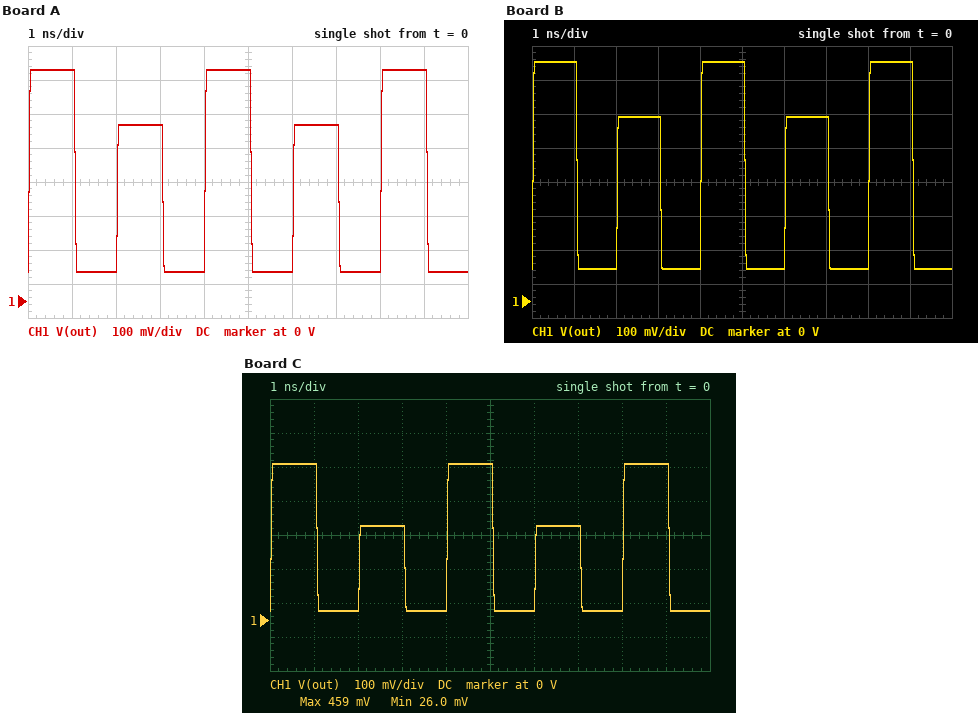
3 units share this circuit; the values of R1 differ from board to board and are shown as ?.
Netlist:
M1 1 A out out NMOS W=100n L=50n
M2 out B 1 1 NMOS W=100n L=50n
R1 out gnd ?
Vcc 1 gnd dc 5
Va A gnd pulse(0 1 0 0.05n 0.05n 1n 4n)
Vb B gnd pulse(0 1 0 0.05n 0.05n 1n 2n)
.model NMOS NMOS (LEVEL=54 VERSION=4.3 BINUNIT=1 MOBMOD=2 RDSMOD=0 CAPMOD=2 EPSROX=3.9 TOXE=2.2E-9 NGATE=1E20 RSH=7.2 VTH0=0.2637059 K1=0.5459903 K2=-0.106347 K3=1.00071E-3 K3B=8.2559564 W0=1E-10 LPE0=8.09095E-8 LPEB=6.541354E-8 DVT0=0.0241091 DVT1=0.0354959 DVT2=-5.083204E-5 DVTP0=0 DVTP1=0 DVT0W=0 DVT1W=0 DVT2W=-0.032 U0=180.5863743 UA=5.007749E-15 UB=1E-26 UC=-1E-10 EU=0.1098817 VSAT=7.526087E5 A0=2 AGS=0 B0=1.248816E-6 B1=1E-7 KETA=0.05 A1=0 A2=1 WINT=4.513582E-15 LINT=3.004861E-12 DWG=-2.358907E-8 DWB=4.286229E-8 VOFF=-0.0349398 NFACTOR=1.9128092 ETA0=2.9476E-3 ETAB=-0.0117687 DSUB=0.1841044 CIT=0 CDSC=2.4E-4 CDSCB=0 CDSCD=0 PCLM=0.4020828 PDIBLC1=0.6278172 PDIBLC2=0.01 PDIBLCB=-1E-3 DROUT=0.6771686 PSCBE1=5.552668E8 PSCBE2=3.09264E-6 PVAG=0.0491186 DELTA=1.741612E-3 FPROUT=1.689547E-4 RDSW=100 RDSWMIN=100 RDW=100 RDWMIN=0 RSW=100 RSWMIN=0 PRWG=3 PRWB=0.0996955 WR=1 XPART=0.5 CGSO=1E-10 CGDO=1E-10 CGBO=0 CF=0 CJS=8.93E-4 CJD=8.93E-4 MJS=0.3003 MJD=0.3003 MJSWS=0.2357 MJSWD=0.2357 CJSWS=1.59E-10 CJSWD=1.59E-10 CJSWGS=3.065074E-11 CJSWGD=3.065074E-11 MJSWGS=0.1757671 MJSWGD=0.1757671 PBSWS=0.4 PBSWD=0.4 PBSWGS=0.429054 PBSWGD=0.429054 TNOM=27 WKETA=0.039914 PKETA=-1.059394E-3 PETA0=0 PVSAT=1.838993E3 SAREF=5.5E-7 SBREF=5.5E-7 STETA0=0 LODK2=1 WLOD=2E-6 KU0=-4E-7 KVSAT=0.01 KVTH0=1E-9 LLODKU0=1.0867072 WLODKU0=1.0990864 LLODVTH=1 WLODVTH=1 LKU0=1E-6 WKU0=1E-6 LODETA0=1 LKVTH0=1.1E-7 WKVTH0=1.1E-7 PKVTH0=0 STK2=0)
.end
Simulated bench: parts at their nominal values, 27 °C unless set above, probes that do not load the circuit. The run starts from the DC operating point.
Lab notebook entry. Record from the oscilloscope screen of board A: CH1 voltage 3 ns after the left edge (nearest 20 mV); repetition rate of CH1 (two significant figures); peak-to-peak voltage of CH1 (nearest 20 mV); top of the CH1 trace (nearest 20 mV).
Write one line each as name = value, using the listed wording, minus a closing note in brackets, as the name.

CH1 voltage 3 ns after the left edge = 520 mV
repetition rate of CH1 = 500 MHz
peak-to-peak voltage of CH1 = 600 mV
top of the CH1 trace = 680 mV
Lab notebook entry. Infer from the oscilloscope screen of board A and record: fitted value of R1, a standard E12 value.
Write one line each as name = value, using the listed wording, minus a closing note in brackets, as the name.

fitted value of R1, a standard E12 value = 1.8 kΩ
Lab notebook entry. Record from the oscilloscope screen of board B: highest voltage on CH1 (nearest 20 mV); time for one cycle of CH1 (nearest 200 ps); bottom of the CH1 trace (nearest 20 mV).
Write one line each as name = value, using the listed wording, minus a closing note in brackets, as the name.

highest voltage on CH1 = 700 mV
time for one cycle of CH1 = 2.0 ns
bottom of the CH1 trace = 100 mV
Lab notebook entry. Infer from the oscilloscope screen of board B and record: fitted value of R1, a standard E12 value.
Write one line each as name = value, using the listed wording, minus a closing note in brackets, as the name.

fitted value of R1, a standard E12 value = 2.2 kΩ
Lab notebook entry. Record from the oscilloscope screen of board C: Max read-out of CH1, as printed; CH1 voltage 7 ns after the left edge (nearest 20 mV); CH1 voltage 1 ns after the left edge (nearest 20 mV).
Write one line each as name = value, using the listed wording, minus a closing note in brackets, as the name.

Max read-out of CH1, as printed = 459 mV
CH1 voltage 7 ns after the left edge = 280 mV
CH1 voltage 1 ns after the left edge = 460 mV
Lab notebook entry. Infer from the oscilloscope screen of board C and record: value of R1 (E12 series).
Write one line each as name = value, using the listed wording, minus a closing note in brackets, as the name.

value of R1 = 330 Ω
